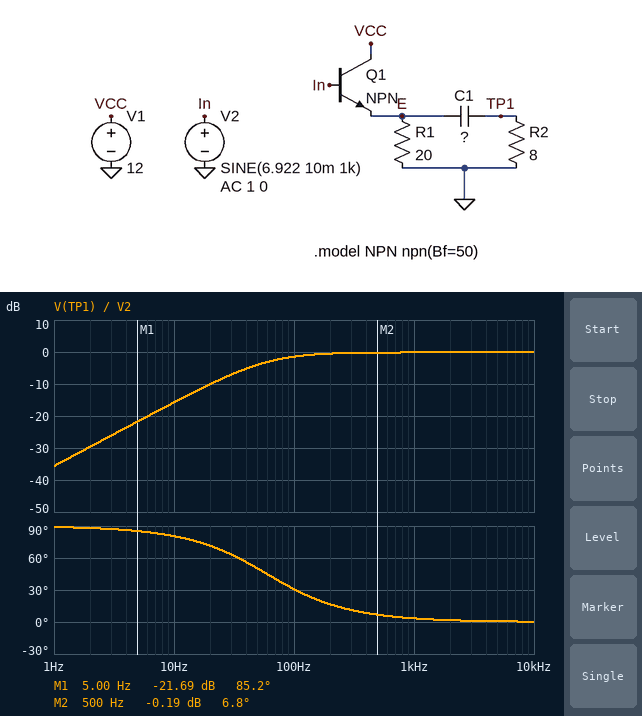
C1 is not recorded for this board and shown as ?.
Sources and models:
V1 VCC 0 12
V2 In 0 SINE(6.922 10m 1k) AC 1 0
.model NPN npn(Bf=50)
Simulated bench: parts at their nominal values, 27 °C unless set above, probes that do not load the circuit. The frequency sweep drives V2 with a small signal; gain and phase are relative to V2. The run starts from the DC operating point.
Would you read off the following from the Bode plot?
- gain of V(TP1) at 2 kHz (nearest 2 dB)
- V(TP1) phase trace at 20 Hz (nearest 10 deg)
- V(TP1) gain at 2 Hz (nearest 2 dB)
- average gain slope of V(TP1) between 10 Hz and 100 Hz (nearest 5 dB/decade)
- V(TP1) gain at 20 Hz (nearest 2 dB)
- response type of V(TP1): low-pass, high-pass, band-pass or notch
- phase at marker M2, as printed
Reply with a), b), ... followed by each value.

a) 0 dB
b) 70 deg
c) -30 dB
d) 15 dB/decade
e) -10 dB
f) high-pass
g) 6.8 deg
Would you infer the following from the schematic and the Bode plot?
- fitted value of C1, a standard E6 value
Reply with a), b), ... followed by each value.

a) 330 µF
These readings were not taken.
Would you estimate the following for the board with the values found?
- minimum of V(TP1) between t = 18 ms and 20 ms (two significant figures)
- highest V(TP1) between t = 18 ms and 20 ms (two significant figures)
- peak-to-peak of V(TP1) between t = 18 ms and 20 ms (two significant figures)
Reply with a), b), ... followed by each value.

a) -9.8 mV
b) 9.8 mV
c) 20 mV
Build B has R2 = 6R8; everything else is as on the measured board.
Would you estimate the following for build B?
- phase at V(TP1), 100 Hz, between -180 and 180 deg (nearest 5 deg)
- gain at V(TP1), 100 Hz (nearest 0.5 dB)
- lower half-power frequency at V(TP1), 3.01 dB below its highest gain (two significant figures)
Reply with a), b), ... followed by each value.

a) 35 deg
b) -2.0 dB
c) 70 Hz
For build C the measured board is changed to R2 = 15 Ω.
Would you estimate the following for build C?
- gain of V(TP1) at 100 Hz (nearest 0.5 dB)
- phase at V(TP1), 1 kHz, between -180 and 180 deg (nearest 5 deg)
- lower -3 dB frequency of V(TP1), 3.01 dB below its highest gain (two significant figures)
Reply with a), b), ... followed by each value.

a) -0.5 dB
b) 0 deg
c) 32 Hz
